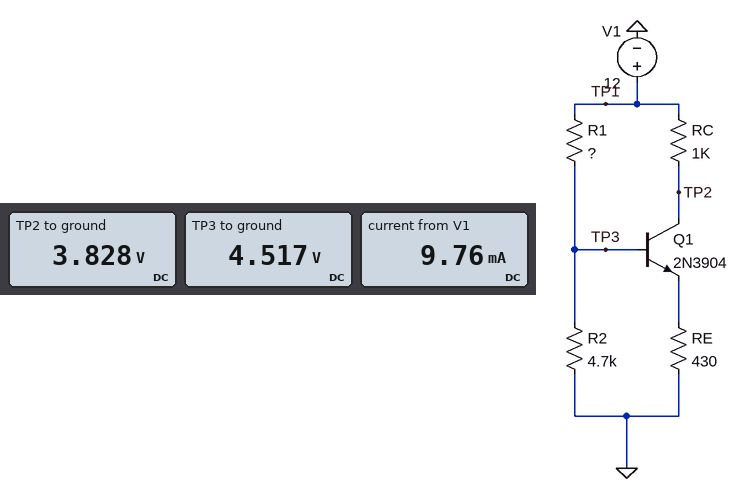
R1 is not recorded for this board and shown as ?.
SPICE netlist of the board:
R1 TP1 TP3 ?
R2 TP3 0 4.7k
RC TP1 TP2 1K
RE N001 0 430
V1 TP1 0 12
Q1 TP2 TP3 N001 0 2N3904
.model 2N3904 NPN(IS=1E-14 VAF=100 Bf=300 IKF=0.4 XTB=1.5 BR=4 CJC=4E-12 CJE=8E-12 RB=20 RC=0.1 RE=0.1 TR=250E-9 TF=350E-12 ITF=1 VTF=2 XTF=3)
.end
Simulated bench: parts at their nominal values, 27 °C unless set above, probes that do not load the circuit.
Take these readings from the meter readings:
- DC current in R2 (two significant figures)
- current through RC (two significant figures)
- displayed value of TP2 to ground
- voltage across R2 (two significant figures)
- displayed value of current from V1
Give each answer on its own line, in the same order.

960 µA
8.2 mA
3.828 V
4.5 V
9.76 mA
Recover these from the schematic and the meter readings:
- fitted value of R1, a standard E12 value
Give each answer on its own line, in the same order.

4.7 kΩ
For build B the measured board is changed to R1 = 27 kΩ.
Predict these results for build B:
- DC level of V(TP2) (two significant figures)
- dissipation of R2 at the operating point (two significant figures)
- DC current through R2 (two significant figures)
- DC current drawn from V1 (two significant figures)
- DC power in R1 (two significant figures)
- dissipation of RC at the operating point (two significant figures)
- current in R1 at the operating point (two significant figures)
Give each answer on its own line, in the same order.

9.5 V
650 µW
370 µA
2.9 mA
3.9 mW
6.2 mW
380 µA
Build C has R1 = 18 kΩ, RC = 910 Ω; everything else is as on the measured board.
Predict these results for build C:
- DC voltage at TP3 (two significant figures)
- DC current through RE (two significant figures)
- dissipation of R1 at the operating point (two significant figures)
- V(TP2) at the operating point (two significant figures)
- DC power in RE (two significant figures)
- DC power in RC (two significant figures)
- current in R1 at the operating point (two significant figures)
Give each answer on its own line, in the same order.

2.4 V
4.1 mA
5.1 mW
8.3 V
7.1 mW
15 mW
530 µA
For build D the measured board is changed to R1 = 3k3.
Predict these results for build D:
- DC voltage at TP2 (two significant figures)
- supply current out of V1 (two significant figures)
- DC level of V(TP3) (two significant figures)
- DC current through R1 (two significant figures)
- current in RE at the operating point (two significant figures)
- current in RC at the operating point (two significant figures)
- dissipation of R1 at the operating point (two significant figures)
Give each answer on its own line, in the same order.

4.0 V
10 mA
4.7 V
2.2 mA
9.2 mA
8.0 mA
16 mW
